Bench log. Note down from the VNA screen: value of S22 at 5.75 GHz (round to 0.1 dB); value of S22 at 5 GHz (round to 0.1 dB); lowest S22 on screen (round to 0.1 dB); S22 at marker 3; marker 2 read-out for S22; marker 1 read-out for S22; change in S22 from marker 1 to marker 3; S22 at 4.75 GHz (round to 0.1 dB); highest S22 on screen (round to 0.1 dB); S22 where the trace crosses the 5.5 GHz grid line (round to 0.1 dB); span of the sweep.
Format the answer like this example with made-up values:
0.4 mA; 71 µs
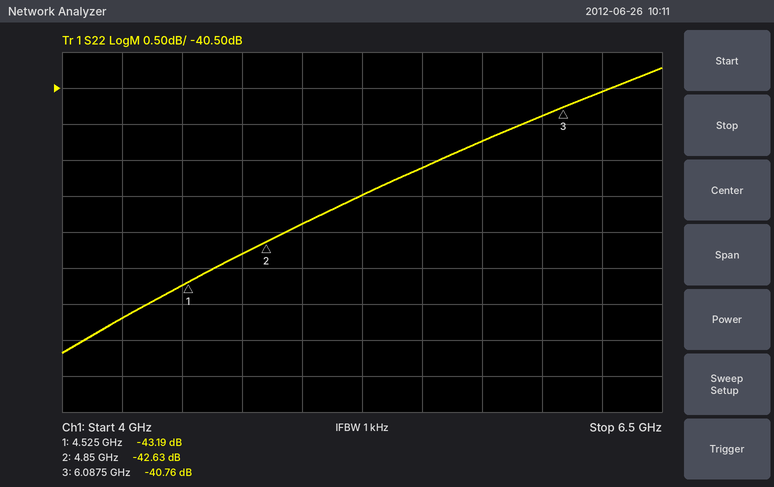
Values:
-41.2 dB; -42.4 dB; -44.2 dB; -40.76 dB; -42.63 dB; -43.19 dB; 2.43 dB; -42.8 dB; -40.2 dB; -41.6 dB; 2.5 GHz
